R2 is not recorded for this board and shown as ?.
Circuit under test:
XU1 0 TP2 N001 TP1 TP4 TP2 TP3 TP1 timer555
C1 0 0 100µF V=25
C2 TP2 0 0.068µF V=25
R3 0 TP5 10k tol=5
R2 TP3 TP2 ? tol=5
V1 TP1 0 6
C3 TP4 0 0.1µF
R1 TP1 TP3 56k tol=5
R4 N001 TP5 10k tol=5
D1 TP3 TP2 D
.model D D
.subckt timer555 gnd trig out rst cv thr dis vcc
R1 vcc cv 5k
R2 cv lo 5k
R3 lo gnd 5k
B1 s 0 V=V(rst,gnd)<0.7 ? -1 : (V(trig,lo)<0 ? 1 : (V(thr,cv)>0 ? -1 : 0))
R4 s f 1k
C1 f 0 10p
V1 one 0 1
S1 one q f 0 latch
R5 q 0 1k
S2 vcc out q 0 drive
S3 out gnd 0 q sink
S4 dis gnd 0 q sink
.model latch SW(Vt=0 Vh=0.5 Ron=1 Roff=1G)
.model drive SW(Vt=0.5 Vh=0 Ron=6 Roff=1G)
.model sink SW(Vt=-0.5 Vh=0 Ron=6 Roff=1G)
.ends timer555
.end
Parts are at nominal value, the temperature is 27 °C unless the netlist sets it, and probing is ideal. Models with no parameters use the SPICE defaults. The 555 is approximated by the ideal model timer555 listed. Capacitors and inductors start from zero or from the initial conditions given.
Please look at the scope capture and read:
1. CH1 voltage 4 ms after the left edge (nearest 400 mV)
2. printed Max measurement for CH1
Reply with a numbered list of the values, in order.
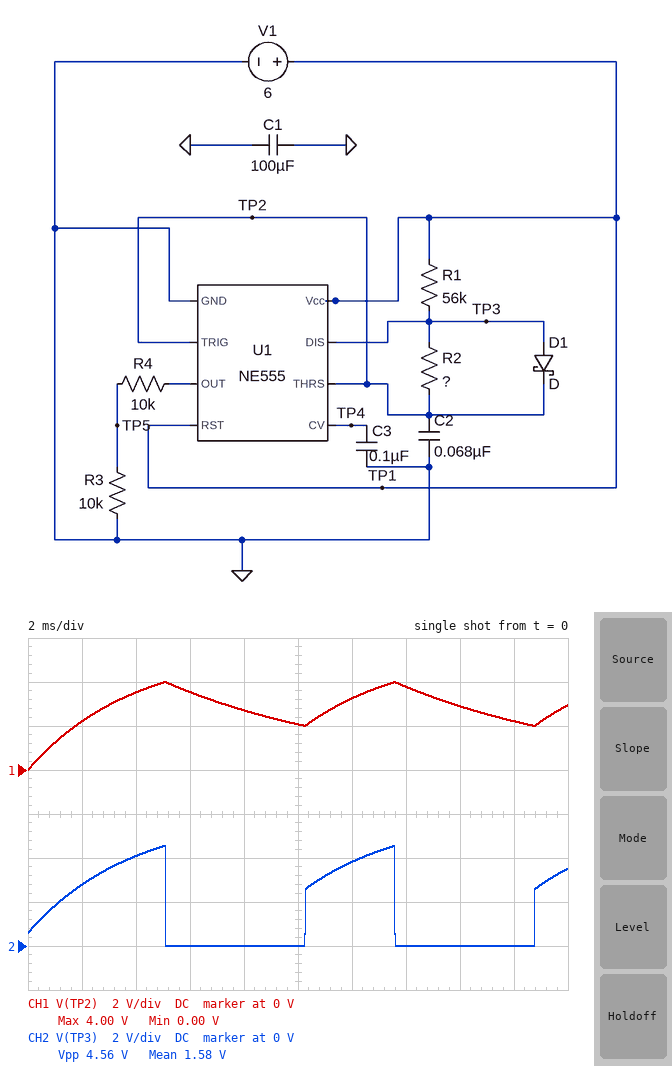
1. 3.6 V
2. 4.00 V
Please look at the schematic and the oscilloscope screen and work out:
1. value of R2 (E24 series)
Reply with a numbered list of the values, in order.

1. 110 kΩ
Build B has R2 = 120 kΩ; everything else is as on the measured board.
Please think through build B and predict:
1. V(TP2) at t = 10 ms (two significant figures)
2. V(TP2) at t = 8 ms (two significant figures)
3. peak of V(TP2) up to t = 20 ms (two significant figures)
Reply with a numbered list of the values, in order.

1. 2.2 V
2. 2.8 V
3. 4.0 V
